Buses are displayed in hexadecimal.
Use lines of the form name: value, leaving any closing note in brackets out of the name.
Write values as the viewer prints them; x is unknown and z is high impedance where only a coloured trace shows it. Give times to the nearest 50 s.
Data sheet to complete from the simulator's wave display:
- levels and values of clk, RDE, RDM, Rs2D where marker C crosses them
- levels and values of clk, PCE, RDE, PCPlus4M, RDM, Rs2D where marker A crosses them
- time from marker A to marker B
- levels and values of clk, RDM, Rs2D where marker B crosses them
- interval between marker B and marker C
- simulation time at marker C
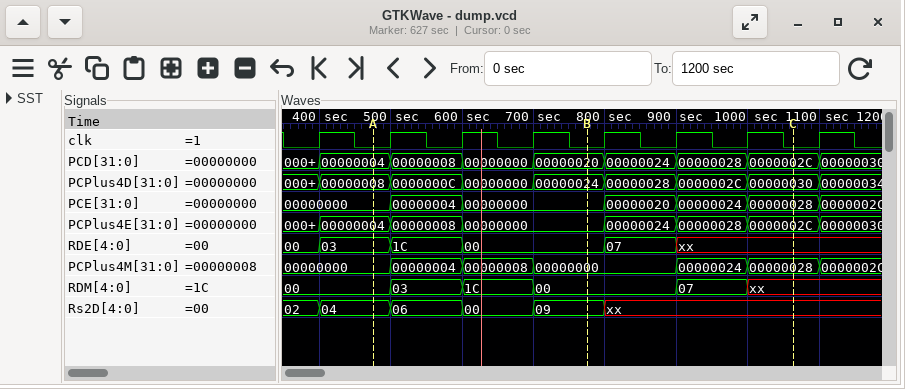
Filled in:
levels and values of clk, RDE, RDM, Rs2D where marker C crosses them: clk=0, RDE=xx, RDM=xx, Rs2D=xx
levels and values of clk, PCE, RDE, PCPlus4M, RDM, Rs2D where marker A crosses them: clk=0, PCE=00000000, RDE=03, PCPlus4M=00000000, RDM=00, Rs2D=04
time from marker A to marker B: 300 s
levels and values of clk, RDM, Rs2D where marker B crosses them: clk=0, RDM=00, Rs2D=09
interval between marker B and marker C: 300 s
simulation time at marker C: 1050 s
